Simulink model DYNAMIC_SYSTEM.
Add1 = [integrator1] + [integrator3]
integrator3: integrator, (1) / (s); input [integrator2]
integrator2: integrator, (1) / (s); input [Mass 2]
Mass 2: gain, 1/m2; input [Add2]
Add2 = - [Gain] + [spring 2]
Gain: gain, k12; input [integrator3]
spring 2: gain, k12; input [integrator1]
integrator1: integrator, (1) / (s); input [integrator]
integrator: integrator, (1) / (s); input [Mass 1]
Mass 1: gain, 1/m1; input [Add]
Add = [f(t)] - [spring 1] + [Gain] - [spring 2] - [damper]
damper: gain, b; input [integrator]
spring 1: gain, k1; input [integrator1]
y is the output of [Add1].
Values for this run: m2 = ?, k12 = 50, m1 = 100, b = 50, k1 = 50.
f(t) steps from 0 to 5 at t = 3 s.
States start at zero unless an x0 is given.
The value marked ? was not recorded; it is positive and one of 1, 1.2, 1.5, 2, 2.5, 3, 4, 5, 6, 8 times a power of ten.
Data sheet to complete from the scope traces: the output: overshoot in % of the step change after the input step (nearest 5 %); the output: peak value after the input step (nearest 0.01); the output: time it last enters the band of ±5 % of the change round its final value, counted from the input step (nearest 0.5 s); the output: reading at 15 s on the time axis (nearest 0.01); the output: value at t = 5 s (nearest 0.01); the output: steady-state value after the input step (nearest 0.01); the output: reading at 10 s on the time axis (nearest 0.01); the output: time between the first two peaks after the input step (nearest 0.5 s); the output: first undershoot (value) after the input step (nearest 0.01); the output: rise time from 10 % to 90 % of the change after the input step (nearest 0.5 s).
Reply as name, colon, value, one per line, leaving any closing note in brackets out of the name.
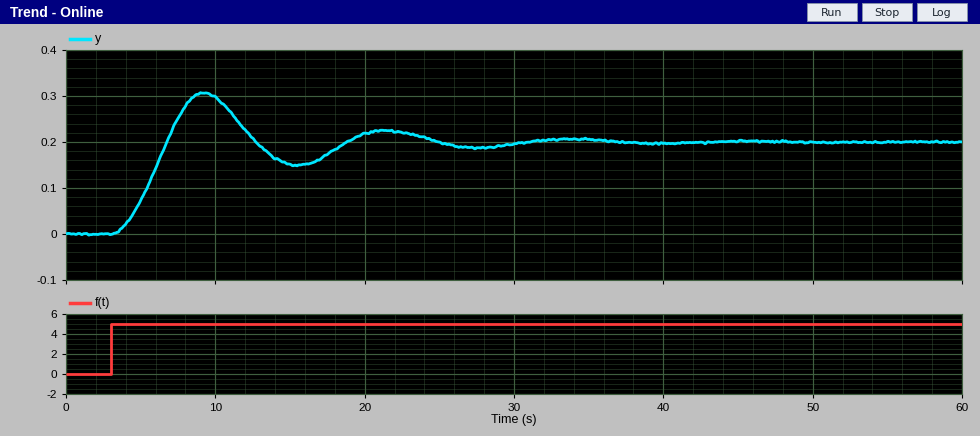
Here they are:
the output: overshoot in % of the step change after the input step: 55 %
the output: peak value after the input step: 0.31
the output: time it last enters the band of ±5 % of the change round its final value, counted from the input step: 26.0 s
the output: reading at 15 s on the time axis: 0.15
the output: value at t = 5 s: 0.07
the output: steady-state value after the input step: 0.20
the output: reading at 10 s on the time axis: 0.30
the output: time between the first two peaks after the input step: 12.0 s
the output: first undershoot (value) after the input step: 0.15
the output: rise time from 10 % to 90 % of the change after the input step: 2.5 s
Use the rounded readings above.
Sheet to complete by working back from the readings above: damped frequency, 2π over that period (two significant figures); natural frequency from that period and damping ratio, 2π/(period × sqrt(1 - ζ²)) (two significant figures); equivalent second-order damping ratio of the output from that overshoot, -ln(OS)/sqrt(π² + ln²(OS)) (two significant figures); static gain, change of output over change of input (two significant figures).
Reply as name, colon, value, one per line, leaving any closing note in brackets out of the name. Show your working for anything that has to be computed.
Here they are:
damped frequency, 2π over that period: 2π / 12 = 0.52 rad/s
natural frequency from that period and damping ratio, 2π/(period × sqrt(1 - ζ²)): 2π / (12 × sqrt(1 - 0.19²)) = 0.53 rad/s
equivalent second-order damping ratio of the output from that overshoot, -ln(OS)/sqrt(π² + ln²(OS)): ln(0.55) = -0.598; 0.598 / sqrt(9.870 + 0.357) = 0.19
static gain, change of output over change of input: (0.2 - 0) / (5 - 0) = 0.040
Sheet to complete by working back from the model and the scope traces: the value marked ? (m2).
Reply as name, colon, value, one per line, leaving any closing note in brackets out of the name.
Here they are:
the value marked ?: 60
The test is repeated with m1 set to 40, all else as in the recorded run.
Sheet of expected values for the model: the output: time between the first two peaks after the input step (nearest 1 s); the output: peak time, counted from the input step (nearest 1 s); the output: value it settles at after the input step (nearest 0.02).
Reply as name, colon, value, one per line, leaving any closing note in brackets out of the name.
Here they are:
the output: time between the first two peaks after the input step: 10 s
the output: peak time, counted from the input step: 6 s
the output: value it settles at after the input step: 0.20
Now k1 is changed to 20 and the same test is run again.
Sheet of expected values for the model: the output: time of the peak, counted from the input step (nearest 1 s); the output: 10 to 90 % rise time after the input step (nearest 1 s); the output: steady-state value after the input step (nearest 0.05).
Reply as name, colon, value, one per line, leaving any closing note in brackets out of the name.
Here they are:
the output: time of the peak, counted from the input step: 10 s
the output: 10 to 90 % rise time after the input step: 4 s
the output: steady-state value after the input step: 0.50
